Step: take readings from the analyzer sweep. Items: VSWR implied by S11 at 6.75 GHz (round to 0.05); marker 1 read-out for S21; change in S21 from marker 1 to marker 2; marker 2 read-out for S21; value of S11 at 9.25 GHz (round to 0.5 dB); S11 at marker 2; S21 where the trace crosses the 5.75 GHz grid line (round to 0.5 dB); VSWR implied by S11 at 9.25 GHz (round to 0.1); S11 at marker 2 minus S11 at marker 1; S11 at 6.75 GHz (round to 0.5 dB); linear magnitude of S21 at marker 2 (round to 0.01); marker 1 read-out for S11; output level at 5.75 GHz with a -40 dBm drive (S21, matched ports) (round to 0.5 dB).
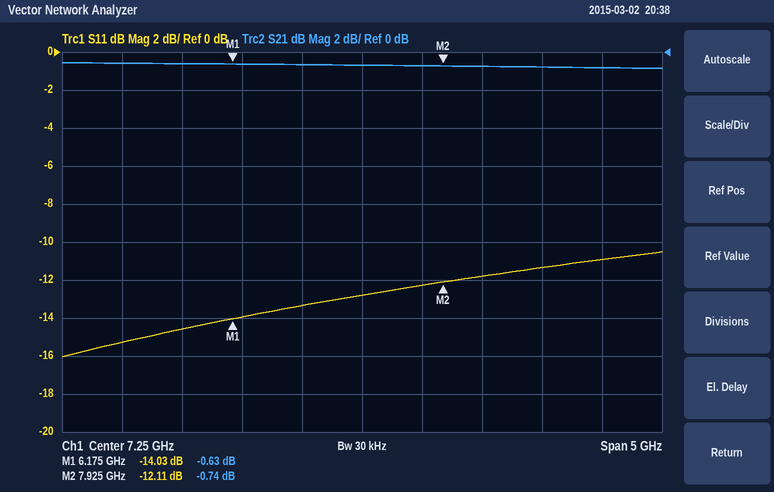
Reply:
1.55
-0.63 dB
-0.11 dB
-0.74 dB
-11.0 dB
-12.11 dB
-0.5 dB
1.8
1.92 dB
-13.5 dB
0.92
-14.03 dB
-40.5 dBm
